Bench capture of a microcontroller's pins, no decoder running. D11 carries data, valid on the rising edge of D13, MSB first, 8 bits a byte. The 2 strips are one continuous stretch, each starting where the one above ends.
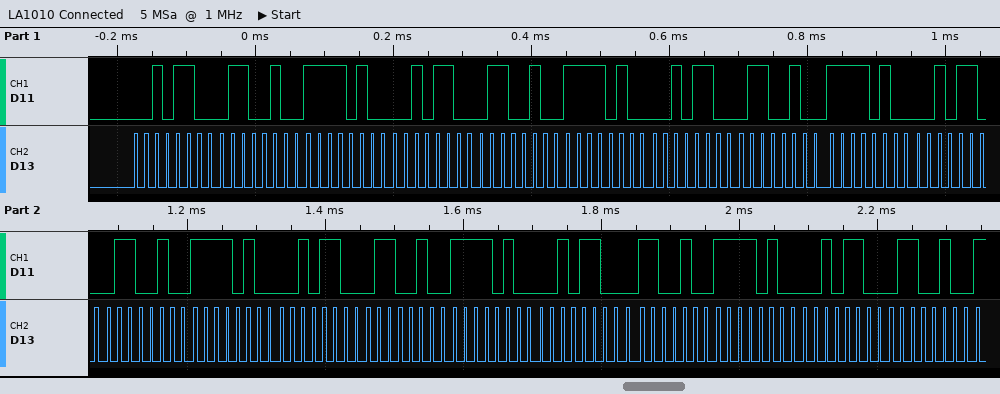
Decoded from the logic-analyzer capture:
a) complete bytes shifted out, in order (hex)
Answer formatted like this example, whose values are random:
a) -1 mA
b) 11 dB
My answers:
a) 0x2C 0x64 0xF4 0x2C 0x64 0xF4 0x2C 0x64 0xF4 0x2C 0x64 0xF4 0x2C 0x64 0xF4 0x2C 0x64 0xF4 0x2C 0x64
